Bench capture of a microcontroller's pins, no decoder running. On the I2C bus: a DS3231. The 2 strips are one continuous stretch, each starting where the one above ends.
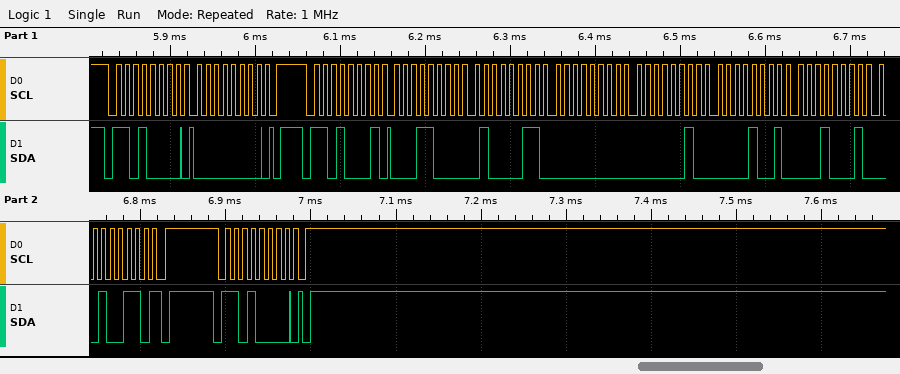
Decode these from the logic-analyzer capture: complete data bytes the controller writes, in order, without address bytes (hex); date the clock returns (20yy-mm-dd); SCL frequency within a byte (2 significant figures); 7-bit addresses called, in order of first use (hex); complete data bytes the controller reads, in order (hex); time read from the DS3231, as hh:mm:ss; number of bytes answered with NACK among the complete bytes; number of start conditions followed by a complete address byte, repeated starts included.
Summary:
00
2026-11-09
100 kHz
0x68
18 43 00 02 09 11 26
00:43:18
1
3
